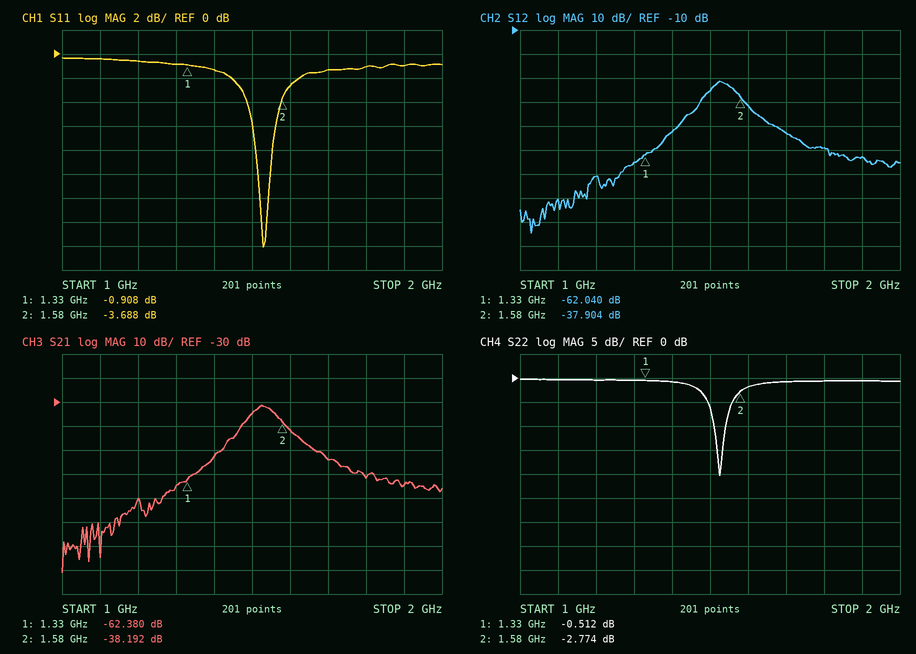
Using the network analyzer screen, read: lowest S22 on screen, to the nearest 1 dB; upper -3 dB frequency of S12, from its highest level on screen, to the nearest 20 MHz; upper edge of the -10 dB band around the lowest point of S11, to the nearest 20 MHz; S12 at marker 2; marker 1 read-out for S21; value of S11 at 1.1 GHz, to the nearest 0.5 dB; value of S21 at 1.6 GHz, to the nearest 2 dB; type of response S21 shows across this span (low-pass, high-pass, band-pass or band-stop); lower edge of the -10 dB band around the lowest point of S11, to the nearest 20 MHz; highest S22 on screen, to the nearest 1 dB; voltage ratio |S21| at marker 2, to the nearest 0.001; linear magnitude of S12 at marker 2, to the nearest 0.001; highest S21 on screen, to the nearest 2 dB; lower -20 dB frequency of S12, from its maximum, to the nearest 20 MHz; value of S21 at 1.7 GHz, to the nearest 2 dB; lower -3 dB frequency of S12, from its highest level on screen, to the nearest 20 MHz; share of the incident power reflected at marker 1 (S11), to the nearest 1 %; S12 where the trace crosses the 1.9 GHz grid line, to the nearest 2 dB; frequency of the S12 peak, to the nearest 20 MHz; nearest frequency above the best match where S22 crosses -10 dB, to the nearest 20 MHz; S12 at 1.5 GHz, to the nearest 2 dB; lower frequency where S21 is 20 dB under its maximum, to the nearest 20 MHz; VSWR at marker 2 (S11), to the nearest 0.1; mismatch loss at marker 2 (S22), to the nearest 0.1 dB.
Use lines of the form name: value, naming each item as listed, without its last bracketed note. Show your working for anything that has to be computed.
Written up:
lowest S22 on screen, to the nearest 1 dB: -20 dB
upper -3 dB frequency of S12, from its highest level on screen, to the nearest 20 MHz: 1.56 GHz
upper edge of the -10 dB band around the lowest point of S11, to the nearest 20 MHz: 1.54 GHz
S12 at marker 2: -37.904 dB
marker 1 read-out for S21: -62.380 dB
value of S11 at 1.1 GHz, to the nearest 0.5 dB: -0.5 dB
value of S21 at 1.6 GHz, to the nearest 2 dB: -42 dB
type of response S21 shows across this span: band-pass
lower edge of the -10 dB band around the lowest point of S11, to the nearest 20 MHz: 1.52 GHz
highest S22 on screen, to the nearest 1 dB: 0 dB
voltage ratio |S21| at marker 2, to the nearest 0.001: 10^(-38.192/20) ≈ 0.012
linear magnitude of S12 at marker 2, to the nearest 0.001: 10^(-37.904/20) ≈ 0.013
highest S21 on screen, to the nearest 2 dB: -32 dB
lower -20 dB frequency of S12, from its maximum, to the nearest 20 MHz: 1.40 GHz
value of S21 at 1.7 GHz, to the nearest 2 dB: -54 dB
lower -3 dB frequency of S12, from its highest level on screen, to the nearest 20 MHz: 1.50 GHz
share of the incident power reflected at marker 1 (S11), to the nearest 1 %: 10^(-0.908/10) ≈ 81 %
S12 where the trace crosses the 1.9 GHz grid line, to the nearest 2 dB: -62 dB
frequency of the S12 peak, to the nearest 20 MHz: 1.52 GHz
nearest frequency above the best match where S22 crosses -10 dB, to the nearest 20 MHz: 1.54 GHz
S12 at 1.5 GHz, to the nearest 2 dB: -36 dB
lower frequency where S21 is 20 dB under its maximum, to the nearest 20 MHz: 1.40 GHz
VSWR at marker 2 (S11), to the nearest 0.1: (1 + 0.6540)/(1 − 0.6540) ≈ 4.8
mismatch loss at marker 2 (S22), to the nearest 0.1 dB: −10 log10(1 − 10^(-2.774/10)) ≈ 3.3 dB
